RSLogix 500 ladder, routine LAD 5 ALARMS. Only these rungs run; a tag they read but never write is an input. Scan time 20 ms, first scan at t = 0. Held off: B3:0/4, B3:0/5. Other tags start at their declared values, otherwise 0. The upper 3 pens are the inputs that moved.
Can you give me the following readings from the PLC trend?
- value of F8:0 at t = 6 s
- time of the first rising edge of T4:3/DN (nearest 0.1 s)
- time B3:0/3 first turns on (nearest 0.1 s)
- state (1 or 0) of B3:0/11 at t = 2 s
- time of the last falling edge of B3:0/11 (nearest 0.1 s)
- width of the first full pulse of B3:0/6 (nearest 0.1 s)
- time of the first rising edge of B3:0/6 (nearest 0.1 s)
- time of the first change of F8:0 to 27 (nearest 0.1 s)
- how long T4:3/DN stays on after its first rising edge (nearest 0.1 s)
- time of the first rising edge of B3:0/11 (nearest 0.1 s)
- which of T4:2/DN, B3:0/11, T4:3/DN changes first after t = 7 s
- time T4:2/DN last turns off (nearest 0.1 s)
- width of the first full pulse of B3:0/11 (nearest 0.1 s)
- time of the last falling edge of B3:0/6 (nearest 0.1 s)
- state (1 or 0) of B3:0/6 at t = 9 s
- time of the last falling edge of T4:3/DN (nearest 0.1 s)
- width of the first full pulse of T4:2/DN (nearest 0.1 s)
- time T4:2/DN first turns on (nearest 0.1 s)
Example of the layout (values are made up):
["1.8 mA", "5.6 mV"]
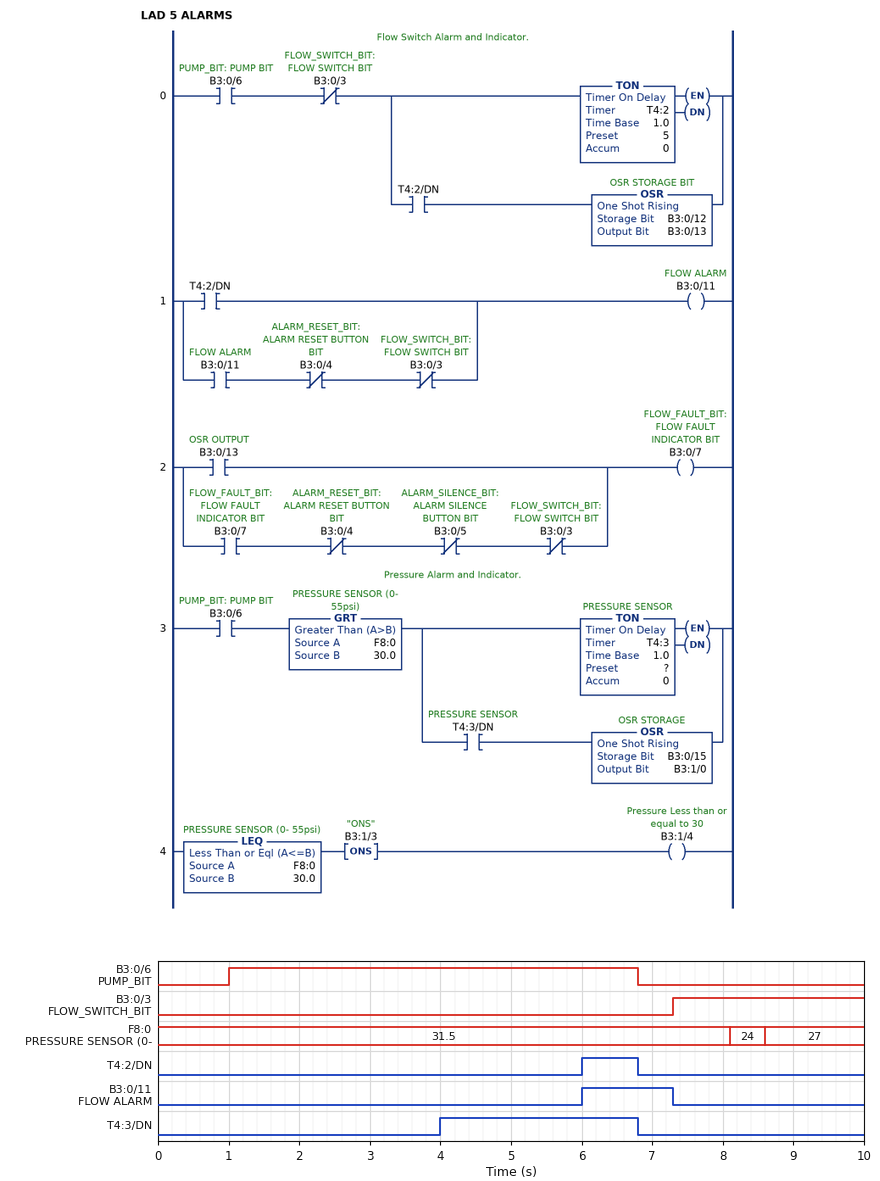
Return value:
["31.5", "4.0 s", "7.3 s", "0", "7.3 s", "5.8 s", "1.0 s", "8.6 s", "2.8 s", "6.0 s", "B3:0/11", "6.8 s", "1.3 s", "6.8 s", "0", "6.8 s", "0.8 s", "6.0 s"]
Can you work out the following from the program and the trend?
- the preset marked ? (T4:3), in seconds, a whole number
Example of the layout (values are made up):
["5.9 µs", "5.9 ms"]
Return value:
["3 s"]
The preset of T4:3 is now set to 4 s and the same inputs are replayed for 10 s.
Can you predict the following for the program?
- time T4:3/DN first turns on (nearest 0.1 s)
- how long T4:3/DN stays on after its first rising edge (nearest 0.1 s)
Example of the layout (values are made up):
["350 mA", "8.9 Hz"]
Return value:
["5.0 s", "1.8 s"]
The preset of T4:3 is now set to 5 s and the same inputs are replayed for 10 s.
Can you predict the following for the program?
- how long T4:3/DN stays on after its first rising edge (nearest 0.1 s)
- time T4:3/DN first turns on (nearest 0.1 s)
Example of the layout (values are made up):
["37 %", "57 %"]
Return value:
["0.8 s", "6.0 s"]
